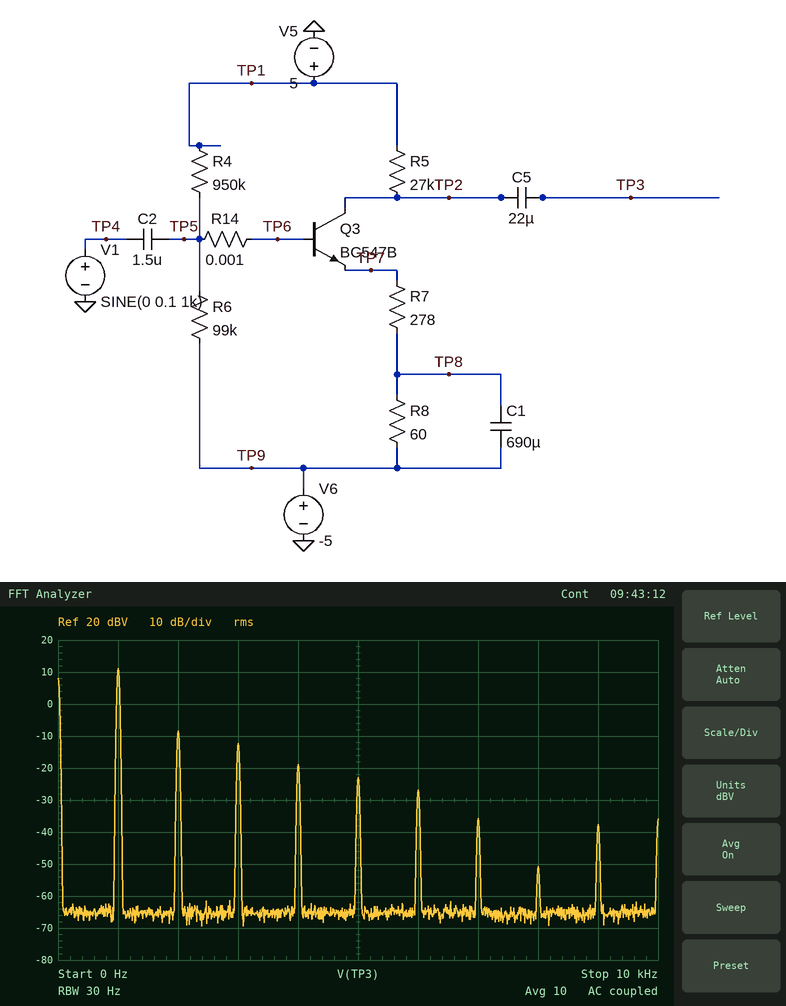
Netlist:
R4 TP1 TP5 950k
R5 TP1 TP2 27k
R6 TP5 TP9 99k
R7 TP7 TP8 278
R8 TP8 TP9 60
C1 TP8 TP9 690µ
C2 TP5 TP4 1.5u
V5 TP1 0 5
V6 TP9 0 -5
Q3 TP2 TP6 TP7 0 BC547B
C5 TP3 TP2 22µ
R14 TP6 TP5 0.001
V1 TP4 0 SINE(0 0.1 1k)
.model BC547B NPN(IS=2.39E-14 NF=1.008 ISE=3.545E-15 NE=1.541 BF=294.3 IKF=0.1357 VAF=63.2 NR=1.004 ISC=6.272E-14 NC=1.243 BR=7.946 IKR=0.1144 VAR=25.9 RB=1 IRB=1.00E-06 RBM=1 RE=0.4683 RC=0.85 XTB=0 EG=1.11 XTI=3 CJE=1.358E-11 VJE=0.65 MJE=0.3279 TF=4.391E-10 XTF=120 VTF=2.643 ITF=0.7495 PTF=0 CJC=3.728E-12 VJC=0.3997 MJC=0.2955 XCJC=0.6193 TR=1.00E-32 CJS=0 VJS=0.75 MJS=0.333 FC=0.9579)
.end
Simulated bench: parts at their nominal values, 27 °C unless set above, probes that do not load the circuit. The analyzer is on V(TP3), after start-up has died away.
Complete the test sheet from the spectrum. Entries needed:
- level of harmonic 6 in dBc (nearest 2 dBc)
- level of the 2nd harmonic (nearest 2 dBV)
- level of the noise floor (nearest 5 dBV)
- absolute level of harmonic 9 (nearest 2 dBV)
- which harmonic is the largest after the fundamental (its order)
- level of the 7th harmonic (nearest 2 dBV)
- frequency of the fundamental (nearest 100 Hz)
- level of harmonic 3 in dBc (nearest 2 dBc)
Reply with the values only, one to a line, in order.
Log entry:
-38 dBc
-8 dBV
-65 dBV
-38 dBV
2
-36 dBV
1.0 kHz
-24 dBc
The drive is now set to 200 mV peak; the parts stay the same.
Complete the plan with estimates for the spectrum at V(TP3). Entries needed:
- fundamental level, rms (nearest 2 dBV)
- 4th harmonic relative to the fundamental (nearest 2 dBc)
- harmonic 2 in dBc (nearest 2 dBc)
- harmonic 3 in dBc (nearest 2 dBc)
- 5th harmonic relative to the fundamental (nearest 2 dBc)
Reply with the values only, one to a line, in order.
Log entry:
12 dBV
-20 dBc
-8 dBc
-36 dBc
-24 dBc
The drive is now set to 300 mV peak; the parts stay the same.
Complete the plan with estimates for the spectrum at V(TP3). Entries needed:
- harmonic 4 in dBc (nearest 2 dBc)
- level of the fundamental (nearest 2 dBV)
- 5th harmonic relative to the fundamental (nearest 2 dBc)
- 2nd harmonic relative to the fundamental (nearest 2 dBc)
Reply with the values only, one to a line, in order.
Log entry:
-24 dBc
10 dBV
-18 dBc
-4 dBc
